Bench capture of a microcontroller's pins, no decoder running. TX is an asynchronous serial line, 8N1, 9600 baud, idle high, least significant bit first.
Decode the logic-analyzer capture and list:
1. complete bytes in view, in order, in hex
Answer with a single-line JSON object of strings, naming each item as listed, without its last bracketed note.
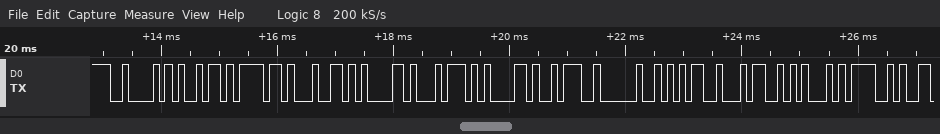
{"complete bytes in view, in order, in hex": "0x42 0x69 0x6F 0x64 0x61 0x74 0x61 0x3A 0x20 0x35 0x34 0x45 0x4F"}
